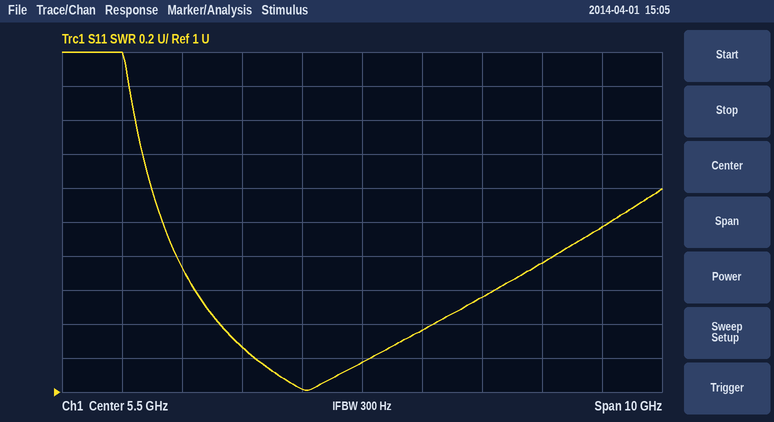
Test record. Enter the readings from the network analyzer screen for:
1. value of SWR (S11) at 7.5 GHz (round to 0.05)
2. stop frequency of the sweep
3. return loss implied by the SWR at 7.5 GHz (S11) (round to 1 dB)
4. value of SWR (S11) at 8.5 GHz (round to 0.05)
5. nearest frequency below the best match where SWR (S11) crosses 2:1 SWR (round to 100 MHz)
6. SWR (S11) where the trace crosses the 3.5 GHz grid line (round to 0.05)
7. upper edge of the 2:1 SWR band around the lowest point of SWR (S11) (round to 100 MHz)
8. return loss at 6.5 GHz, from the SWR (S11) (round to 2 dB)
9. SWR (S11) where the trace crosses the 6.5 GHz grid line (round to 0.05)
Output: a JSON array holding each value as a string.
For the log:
["1.55", "10.5 GHz", "13 dB", "1.75", "2.2 GHz", "1.25", "9.6 GHz", "16 dB", "1.35"]
